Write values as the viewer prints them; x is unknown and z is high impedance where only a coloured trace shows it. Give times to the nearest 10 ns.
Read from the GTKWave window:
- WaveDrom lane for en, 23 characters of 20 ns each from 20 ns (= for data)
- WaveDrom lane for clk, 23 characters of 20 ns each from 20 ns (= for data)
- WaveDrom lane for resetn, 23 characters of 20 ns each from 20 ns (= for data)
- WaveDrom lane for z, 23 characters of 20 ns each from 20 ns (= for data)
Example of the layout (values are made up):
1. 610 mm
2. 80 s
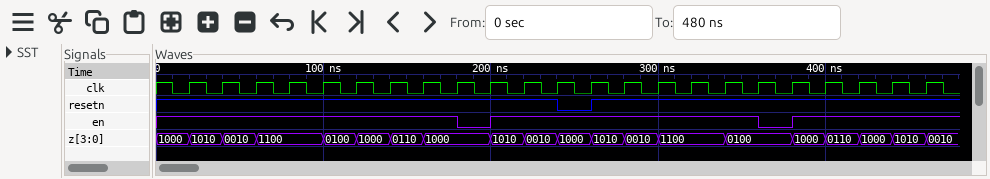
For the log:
1. {name: 'en', wave: '1.......01.......01....'}
2. {name: 'clk', wave: 'p......................'}
3. {name: 'resetn', wave: '1..........01..........'}
4. {name: 'z', wave: '===.====.======.=.=====', data: '1010 0010 1100 0100 1000 0110 1000 1010 0010 1000 1010 0010 1100 0100 1000 0110 1000 1010 0010'}
